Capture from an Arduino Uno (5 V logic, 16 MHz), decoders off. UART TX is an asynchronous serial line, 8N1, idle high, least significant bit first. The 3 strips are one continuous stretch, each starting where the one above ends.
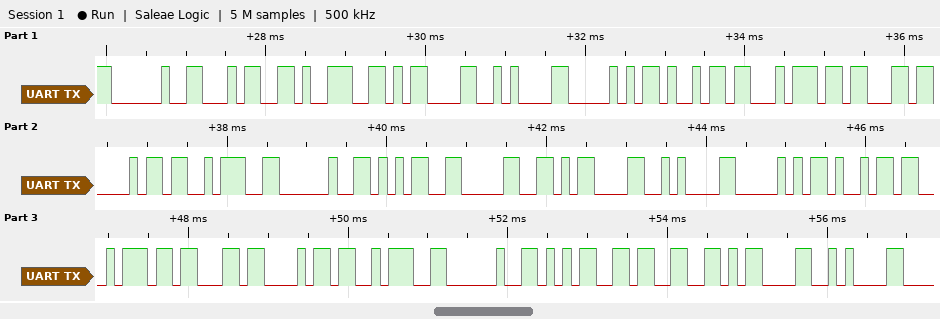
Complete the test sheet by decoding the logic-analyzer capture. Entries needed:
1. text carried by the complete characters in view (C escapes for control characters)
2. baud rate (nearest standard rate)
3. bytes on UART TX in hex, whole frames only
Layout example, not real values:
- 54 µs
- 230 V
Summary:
- " 49\r\nPitch: 50\r\nPitch: 53\r\n"
- 9600 baud
- 20 34 39 0D 0A 50 69 74 63 68 3A 20 35 30 0D 0A 50 69 74 63 68 3A 20 35 33 0D 0A
